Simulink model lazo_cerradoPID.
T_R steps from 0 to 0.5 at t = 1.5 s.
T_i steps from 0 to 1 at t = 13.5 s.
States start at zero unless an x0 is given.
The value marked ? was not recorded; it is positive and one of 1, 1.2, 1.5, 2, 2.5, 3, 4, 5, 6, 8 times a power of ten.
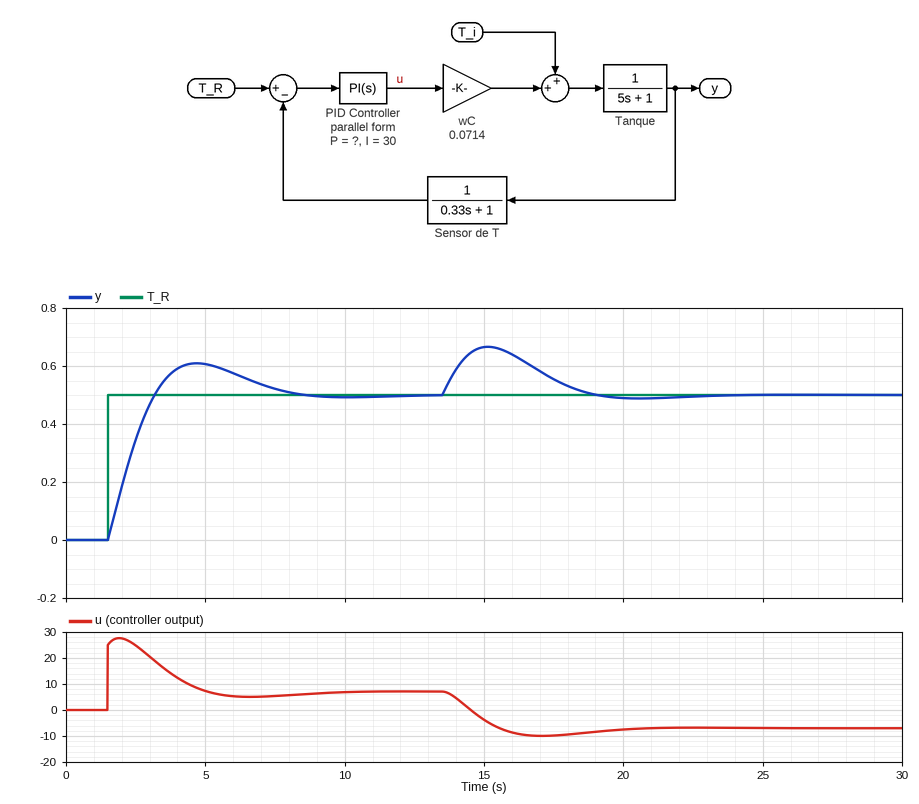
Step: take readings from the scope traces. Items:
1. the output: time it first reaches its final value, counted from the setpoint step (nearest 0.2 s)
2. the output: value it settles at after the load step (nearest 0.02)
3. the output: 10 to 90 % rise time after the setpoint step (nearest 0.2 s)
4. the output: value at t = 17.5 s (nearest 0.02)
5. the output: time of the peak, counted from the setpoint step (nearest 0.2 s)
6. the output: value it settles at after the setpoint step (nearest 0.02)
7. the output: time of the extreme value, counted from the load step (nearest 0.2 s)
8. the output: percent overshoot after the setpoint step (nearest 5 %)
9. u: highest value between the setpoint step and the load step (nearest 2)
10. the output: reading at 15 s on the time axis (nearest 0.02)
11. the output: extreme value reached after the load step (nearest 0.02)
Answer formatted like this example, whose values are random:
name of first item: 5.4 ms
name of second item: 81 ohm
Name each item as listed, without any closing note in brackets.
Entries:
the output: time it first reaches its final value, counted from the setpoint step: 1.6 s
the output: value it settles at after the load step: 0.50
the output: 10 to 90 % rise time after the setpoint step: 1.2 s
the output: value at t = 17.5 s: 0.56
the output: time of the peak, counted from the setpoint step: 3.2 s
the output: value it settles at after the setpoint step: 0.50
the output: time of the extreme value, counted from the load step: 1.6 s
the output: percent overshoot after the setpoint step: 20 %
u: highest value between the setpoint step and the load step: 28
the output: reading at 15 s on the time axis: 0.66
the output: extreme value reached after the load step: 0.66
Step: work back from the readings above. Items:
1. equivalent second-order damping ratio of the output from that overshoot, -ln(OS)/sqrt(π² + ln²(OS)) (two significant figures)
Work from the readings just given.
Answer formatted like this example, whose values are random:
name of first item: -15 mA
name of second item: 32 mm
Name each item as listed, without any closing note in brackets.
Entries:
equivalent second-order damping ratio of the output from that overshoot, -ln(OS)/sqrt(π² + ln²(OS)): 0.46
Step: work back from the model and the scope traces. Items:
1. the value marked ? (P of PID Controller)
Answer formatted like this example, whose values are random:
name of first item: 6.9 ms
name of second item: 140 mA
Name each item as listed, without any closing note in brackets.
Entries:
the value marked ?: 50
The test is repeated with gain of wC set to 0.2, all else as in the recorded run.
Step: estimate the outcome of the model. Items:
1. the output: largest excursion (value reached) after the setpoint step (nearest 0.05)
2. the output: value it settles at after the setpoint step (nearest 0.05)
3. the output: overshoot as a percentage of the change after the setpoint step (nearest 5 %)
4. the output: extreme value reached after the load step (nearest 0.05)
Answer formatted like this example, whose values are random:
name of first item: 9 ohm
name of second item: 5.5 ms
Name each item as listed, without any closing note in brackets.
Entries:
the output: largest excursion (value reached) after the setpoint step: 0.65
the output: value it settles at after the setpoint step: 0.50
the output: overshoot as a percentage of the change after the setpoint step: 35 %
the output: extreme value reached after the load step: 0.60
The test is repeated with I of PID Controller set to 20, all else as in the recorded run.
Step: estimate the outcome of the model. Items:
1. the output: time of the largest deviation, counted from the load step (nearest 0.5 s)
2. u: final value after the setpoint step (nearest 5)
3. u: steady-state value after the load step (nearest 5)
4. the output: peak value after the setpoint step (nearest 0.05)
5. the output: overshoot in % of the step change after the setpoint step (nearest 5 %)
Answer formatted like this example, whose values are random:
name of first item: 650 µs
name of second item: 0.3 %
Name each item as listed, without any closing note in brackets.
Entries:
the output: time of the largest deviation, counted from the load step: 2.0 s
u: final value after the setpoint step: 5
u: steady-state value after the load step: -5
the output: peak value after the setpoint step: 0.55
the output: overshoot in % of the step change after the setpoint step: 10 %
